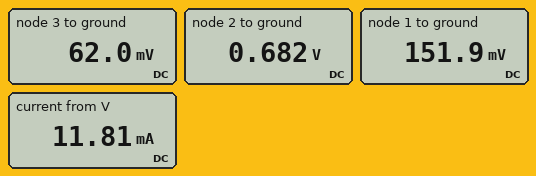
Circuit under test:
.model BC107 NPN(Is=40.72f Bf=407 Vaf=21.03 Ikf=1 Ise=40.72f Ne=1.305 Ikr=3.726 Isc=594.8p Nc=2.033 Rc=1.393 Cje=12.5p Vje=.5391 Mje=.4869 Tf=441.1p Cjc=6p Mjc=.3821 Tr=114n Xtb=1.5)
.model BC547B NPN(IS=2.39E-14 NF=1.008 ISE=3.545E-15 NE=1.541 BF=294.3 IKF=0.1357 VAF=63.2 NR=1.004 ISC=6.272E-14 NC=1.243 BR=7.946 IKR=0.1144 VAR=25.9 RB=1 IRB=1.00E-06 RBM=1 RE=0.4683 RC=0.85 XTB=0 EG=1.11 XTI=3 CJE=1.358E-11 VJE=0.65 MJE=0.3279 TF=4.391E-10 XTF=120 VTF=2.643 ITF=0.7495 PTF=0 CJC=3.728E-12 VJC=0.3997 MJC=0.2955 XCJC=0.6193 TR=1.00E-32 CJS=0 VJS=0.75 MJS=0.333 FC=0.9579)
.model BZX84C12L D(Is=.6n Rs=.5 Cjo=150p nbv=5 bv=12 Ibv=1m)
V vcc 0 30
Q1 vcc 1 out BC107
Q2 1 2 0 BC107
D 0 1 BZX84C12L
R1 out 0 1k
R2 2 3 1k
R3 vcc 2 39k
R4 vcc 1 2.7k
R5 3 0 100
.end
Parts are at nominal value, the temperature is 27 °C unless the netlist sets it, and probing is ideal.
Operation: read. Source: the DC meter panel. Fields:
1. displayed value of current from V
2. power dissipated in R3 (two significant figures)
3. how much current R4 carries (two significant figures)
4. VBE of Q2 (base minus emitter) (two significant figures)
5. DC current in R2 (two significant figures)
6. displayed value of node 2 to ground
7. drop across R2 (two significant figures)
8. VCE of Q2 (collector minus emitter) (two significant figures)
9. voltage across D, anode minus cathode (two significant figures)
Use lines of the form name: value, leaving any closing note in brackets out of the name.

displayed value of current from V: 11.81 mA
power dissipated in R3: 22 mW
how much current R4 carries: 11 mA
VBE of Q2 (base minus emitter): 680 mV
DC current in R2: 620 µA
displayed value of node 2 to ground: 0.682 V
drop across R2: 620 mV
VCE of Q2 (collector minus emitter): 150 mV
voltage across D, anode minus cathode: -150 mV
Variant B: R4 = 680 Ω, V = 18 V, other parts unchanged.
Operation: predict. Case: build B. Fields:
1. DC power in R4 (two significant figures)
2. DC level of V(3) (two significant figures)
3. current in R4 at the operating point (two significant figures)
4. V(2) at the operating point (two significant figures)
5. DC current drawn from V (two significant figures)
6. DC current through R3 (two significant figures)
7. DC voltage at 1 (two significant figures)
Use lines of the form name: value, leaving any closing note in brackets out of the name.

DC power in R4: 48 mW
DC level of V(3): 45 mV
current in R4 at the operating point: 8.4 mA
V(2) at the operating point: 490 mV
DC current drawn from V: 20 mA
DC current through R3: 450 µA
DC voltage at 1: 12 V
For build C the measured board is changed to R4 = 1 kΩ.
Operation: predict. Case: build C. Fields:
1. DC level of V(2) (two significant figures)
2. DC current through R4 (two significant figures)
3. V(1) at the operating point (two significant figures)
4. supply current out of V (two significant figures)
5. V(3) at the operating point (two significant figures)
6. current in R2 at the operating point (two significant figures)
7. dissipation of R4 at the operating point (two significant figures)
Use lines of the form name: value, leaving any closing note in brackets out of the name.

DC level of V(2): 700 mV
DC current through R4: 28 mA
V(1) at the operating point: 2.2 V
supply current out of V: 30 mA
V(3) at the operating point: 64 mV
current in R2 at the operating point: 640 µA
dissipation of R4 at the operating point: 770 mW
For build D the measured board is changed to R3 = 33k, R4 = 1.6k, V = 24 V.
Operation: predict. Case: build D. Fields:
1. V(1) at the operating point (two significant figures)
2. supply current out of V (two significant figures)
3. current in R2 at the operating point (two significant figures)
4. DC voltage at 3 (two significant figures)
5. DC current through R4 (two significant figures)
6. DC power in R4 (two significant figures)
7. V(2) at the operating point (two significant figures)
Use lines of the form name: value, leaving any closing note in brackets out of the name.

V(1) at the operating point: 230 mV
supply current out of V: 16 mA
current in R2 at the operating point: 630 µA
DC voltage at 3: 63 mV
DC current through R4: 15 mA
DC power in R4: 350 mW
V(2) at the operating point: 690 mV
